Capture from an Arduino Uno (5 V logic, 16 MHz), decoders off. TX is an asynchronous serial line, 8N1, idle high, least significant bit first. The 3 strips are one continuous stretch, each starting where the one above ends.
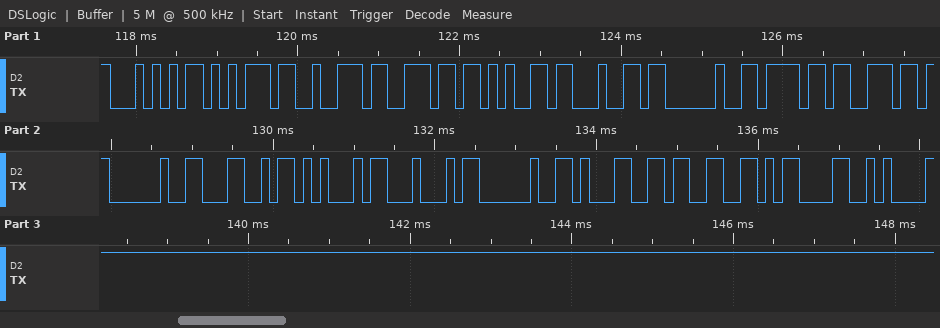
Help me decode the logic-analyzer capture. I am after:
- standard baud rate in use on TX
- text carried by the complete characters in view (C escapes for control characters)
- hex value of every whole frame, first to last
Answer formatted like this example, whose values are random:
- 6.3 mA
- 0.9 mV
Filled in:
- 9600 baud
- "Turned on LED 13\r\n"
- 54 75 72 6E 65 64 20 6F 6E 20 4C 45 44 20 31 33 0D 0A
